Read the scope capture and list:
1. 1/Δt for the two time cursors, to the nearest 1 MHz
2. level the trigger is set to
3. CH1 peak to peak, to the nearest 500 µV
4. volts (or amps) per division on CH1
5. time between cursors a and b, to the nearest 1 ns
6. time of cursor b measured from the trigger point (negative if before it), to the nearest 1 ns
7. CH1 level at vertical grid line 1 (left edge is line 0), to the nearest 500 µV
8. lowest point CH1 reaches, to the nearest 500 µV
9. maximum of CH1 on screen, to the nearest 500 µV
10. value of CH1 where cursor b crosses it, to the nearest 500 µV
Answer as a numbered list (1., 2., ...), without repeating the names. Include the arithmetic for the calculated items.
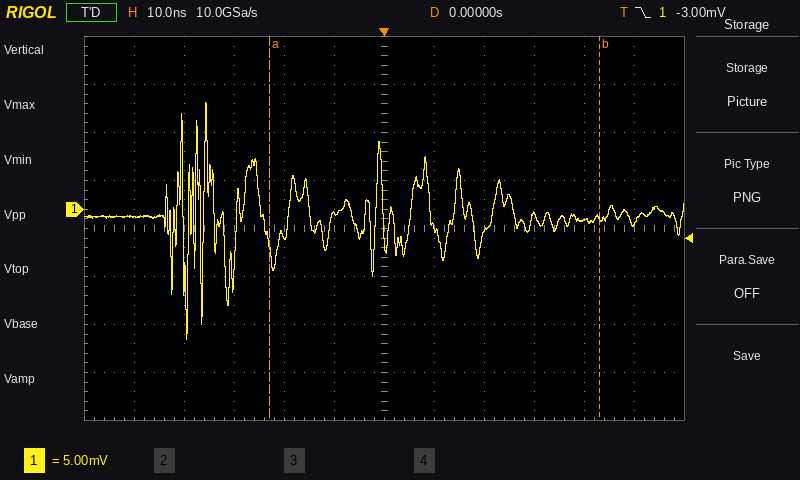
1. 1 / 66 ns ≈ 15 MHz
2. -3.00 mV
3. 11.0 mV − (-13.5 mV) = 24.5 mV
4. 5 mV
5. 66 ns
6. +43 ns
7. -1.0 mV
8. -13.5 mV
9. 11.0 mV
10. -1.0 mV
